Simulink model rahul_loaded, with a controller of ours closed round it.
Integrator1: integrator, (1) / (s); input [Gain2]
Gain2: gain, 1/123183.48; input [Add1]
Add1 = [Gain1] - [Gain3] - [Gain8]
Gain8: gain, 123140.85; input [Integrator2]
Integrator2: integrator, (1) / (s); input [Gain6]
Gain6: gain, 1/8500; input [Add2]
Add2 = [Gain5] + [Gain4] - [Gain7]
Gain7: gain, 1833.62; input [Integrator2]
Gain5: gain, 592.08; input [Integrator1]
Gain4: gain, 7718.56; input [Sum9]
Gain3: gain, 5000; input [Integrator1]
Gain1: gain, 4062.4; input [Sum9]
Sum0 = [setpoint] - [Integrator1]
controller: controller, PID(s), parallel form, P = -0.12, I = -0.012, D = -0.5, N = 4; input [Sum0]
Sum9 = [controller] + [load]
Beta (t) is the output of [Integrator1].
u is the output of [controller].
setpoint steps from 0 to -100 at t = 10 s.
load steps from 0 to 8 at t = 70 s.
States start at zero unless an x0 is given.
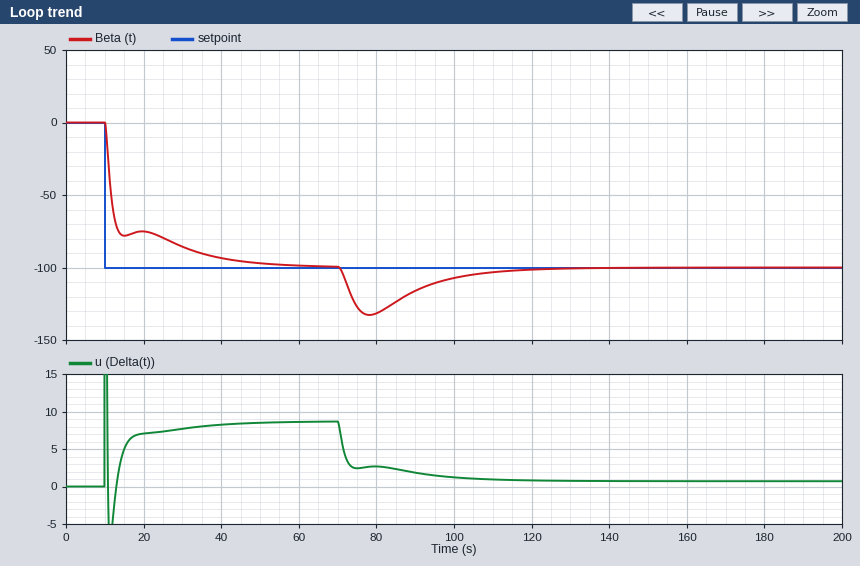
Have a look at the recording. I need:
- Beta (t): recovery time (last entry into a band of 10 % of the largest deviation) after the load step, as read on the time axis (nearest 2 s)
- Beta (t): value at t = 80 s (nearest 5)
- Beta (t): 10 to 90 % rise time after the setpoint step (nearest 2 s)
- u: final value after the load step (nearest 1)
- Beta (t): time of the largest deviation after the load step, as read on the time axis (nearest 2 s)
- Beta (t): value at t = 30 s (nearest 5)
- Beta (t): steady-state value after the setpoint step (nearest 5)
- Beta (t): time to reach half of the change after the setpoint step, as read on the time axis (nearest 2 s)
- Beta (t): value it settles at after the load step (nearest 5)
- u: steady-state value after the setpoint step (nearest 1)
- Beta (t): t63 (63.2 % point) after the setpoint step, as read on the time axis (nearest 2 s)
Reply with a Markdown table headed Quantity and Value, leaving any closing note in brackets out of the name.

| Quantity | Value |
|---|---|
| Beta (t): recovery time (last entry into a band of 10 % of the largest deviation) after the load step, as read on the time axis | 110 s |
| Beta (t): value at t = 80 s | -130 |
| Beta (t): 10 to 90 % rise time after the setpoint step | 24 s |
| u: final value after the load step | 1 |
| Beta (t): time of the largest deviation after the load step, as read on the time axis | 78 s |
| Beta (t): value at t = 30 s | -85 |
| Beta (t): steady-state value after the setpoint step | -100 |
| Beta (t): time to reach half of the change after the setpoint step, as read on the time axis | 12 s |
| Beta (t): value it settles at after the load step | -100 |
| u: steady-state value after the setpoint step | 9 |
| Beta (t): t63 (63.2 % point) after the setpoint step, as read on the time axis | 12 s |
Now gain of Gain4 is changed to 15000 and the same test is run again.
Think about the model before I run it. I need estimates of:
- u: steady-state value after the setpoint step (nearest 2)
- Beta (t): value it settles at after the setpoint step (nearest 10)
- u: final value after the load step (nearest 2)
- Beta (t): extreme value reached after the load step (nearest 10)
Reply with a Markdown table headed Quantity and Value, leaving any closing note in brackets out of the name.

| Quantity | Value |
|---|---|
| u: steady-state value after the setpoint step | 4 |
| Beta (t): value it settles at after the setpoint step | -100 |
| u: final value after the load step | -4 |
| Beta (t): extreme value reached after the load step | -140 |
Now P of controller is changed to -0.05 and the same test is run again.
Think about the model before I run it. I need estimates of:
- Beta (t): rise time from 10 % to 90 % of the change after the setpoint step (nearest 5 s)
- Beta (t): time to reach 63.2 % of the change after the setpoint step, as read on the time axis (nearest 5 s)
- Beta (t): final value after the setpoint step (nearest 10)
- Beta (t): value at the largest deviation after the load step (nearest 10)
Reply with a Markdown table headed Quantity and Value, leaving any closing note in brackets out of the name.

| Quantity | Value |
|---|---|
| Beta (t): rise time from 10 % to 90 % of the change after the setpoint step | 20 s |
| Beta (t): time to reach 63.2 % of the change after the setpoint step, as read on the time axis | 15 s |
| Beta (t): final value after the setpoint step | -100 |
| Beta (t): value at the largest deviation after the load step | -140 |
